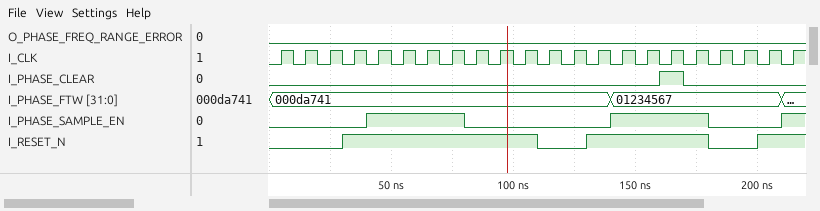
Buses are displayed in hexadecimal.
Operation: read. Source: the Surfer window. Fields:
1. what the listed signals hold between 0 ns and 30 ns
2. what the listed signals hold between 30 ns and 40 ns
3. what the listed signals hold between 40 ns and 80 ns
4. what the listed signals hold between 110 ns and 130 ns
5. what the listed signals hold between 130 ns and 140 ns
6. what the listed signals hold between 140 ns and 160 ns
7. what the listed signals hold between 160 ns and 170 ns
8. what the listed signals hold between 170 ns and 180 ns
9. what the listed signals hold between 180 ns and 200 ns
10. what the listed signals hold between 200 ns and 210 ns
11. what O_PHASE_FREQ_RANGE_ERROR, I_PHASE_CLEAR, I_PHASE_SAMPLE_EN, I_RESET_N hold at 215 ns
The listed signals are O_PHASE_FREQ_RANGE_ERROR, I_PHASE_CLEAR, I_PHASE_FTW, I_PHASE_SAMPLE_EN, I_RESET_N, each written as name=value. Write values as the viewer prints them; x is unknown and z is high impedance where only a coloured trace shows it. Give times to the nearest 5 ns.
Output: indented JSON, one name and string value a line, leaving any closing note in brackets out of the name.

{
  "what the listed signals hold between 0 ns and 30 ns": "O_PHASE_FREQ_RANGE_ERROR=0, I_PHASE_CLEAR=0, I_PHASE_FTW=000da741, I_PHASE_SAMPLE_EN=0, I_RESET_N=0",
  "what the listed signals hold between 30 ns and 40 ns": "O_PHASE_FREQ_RANGE_ERROR=0, I_PHASE_CLEAR=0, I_PHASE_FTW=000da741, I_PHASE_SAMPLE_EN=0, I_RESET_N=1",
  "what the listed signals hold between 40 ns and 80 ns": "O_PHASE_FREQ_RANGE_ERROR=0, I_PHASE_CLEAR=0, I_PHASE_FTW=000da741, I_PHASE_SAMPLE_EN=1, I_RESET_N=1",
  "what the listed signals hold between 110 ns and 130 ns": "O_PHASE_FREQ_RANGE_ERROR=0, I_PHASE_CLEAR=0, I_PHASE_FTW=000da741, I_PHASE_SAMPLE_EN=0, I_RESET_N=0",
  "what the listed signals hold between 130 ns and 140 ns": "O_PHASE_FREQ_RANGE_ERROR=0, I_PHASE_CLEAR=0, I_PHASE_FTW=000da741, I_PHASE_SAMPLE_EN=0, I_RESET_N=1",
  "what the listed signals hold between 140 ns and 160 ns": "O_PHASE_FREQ_RANGE_ERROR=0, I_PHASE_CLEAR=0, I_PHASE_FTW=01234567, I_PHASE_SAMPLE_EN=1, I_RESET_N=1",
  "what the listed signals hold between 160 ns and 170 ns": "O_PHASE_FREQ_RANGE_ERROR=0, I_PHASE_CLEAR=1, I_PHASE_FTW=01234567, I_PHASE_SAMPLE_EN=1, I_RESET_N=1",
  "what the listed signals hold between 170 ns and 180 ns": "O_PHASE_FREQ_RANGE_ERROR=0, I_PHASE_CLEAR=0, I_PHASE_FTW=01234567, I_PHASE_SAMPLE_EN=1, I_RESET_N=1",
  "what the listed signals hold between 180 ns and 200 ns": "O_PHASE_FREQ_RANGE_ERROR=0, I_PHASE_CLEAR=0, I_PHASE_FTW=01234567, I_PHASE_SAMPLE_EN=0, I_RESET_N=0",
  "what the listed signals hold between 200 ns and 210 ns": "O_PHASE_FREQ_RANGE_ERROR=0, I_PHASE_CLEAR=0, I_PHASE_FTW=01234567, I_PHASE_SAMPLE_EN=0, I_RESET_N=1",
  "what O_PHASE_FREQ_RANGE_ERROR, I_PHASE_CLEAR, I_PHASE_SAMPLE_EN, I_RESET_N hold at 215 ns": "O_PHASE_FREQ_RANGE_ERROR=0, I_PHASE_CLEAR=0, I_PHASE_SAMPLE_EN=1, I_RESET_N=1"
}
